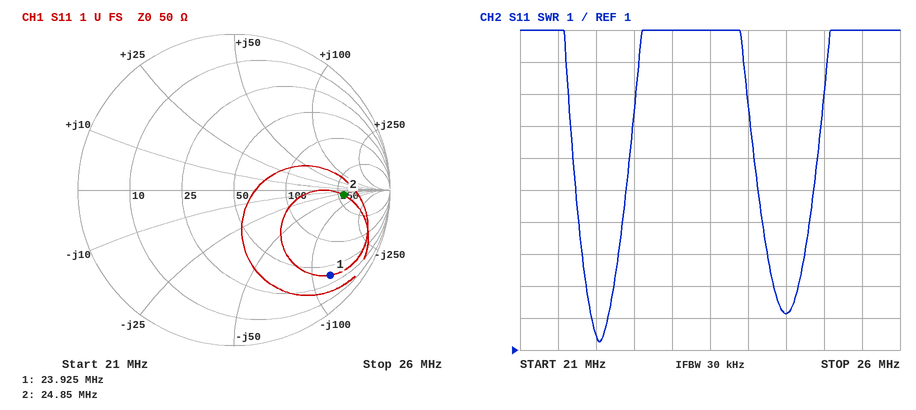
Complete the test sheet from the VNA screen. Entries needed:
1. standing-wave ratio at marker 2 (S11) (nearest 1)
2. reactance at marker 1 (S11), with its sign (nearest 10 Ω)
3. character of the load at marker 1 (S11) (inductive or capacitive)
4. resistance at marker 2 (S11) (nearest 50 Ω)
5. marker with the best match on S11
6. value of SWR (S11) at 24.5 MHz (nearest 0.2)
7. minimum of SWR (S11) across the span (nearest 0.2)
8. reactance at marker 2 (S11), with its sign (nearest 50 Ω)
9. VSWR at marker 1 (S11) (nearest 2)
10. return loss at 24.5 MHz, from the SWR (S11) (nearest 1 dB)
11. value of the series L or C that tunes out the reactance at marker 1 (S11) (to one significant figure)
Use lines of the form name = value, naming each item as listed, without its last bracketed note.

standing-wave ratio at marker 2 (S11) = 6
reactance at marker 1 (S11), with its sign = -120 Ω
character of the load at marker 1 (S11) = capacitive
resistance at marker 2 (S11) = 300 Ω
marker with the best match on S11 = marker 2
value of SWR (S11) at 24.5 MHz = 2.2
minimum of SWR (S11) across the span = 1.2
reactance at marker 2 (S11), with its sign = -50 Ω
VSWR at marker 1 (S11) = 10
return loss at 24.5 MHz, from the SWR (S11) = 9 dB
value of the series L or C that tunes out the reactance at marker 1 (S11) = 800 nH
